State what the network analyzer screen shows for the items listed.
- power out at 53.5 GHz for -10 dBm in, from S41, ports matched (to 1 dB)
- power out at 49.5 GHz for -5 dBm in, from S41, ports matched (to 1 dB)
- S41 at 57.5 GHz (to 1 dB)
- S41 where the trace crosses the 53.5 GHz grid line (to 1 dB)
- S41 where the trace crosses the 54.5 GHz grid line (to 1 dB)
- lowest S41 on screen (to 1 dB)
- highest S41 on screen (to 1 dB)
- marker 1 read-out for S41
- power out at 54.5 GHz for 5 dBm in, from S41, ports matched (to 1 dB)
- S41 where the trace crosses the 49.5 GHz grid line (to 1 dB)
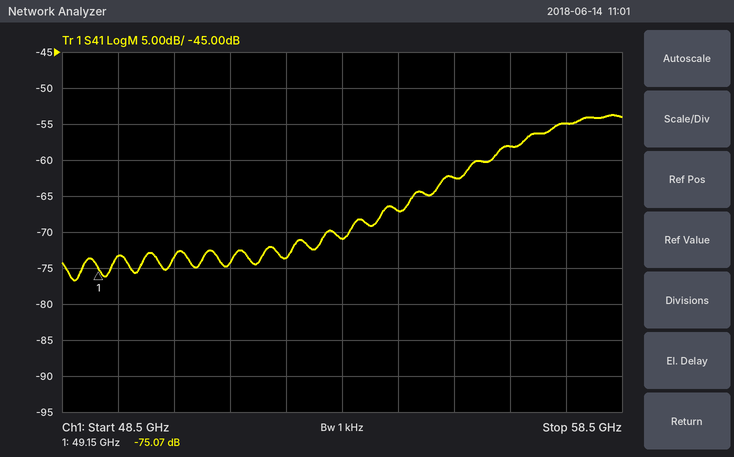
-81 dBm
-78 dBm
-55 dB
-71 dB
-67 dB
-77 dB
-54 dB
-75.07 dB
-62 dBm
-73 dB
